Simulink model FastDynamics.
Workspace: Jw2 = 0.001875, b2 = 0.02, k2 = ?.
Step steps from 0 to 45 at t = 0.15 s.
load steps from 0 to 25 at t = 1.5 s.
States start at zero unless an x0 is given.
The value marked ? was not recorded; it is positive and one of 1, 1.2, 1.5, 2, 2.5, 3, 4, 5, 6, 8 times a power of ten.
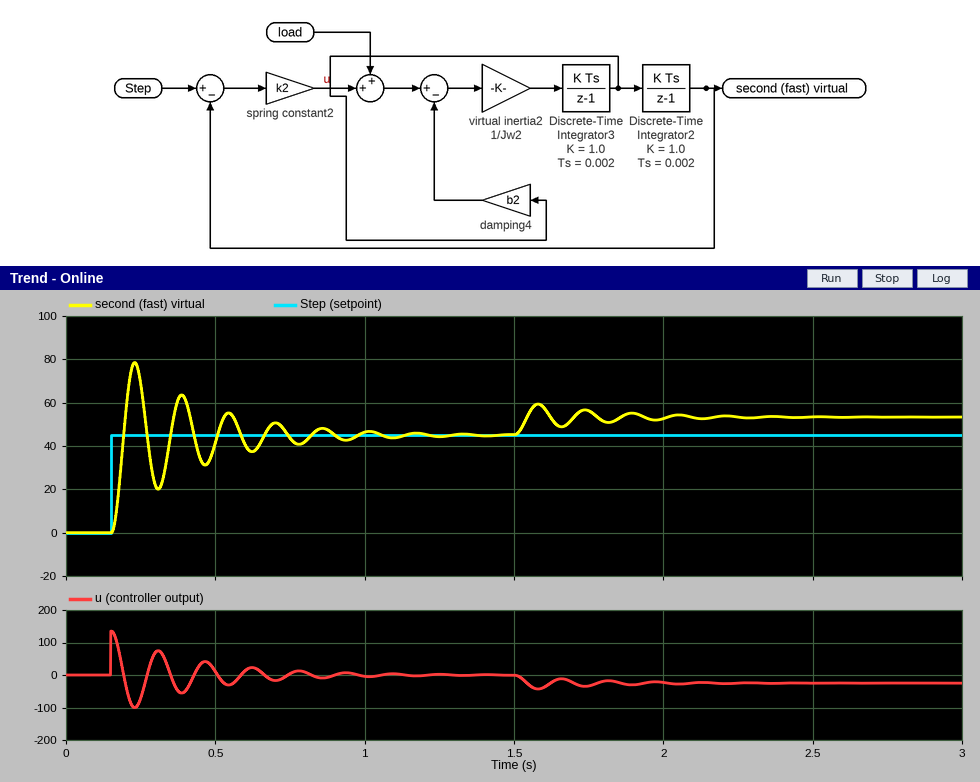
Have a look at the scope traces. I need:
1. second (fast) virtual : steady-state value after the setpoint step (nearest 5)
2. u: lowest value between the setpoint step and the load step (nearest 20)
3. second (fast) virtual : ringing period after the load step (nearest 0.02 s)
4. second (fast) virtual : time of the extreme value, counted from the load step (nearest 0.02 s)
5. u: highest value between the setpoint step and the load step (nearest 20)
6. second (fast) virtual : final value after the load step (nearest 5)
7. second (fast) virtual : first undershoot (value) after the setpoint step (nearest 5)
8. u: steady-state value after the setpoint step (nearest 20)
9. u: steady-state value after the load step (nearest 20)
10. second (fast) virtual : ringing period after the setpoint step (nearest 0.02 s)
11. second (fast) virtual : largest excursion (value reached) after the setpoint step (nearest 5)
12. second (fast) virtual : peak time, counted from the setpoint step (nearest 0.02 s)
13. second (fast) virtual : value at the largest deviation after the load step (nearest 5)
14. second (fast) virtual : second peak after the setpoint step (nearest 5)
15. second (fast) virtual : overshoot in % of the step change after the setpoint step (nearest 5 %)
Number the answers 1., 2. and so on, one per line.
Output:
1. 45
2. -100
3. 0.16 s
4. 0.08 s
5. 140
6. 55
7. 20
8. 0
9. -20
10. 0.16 s
11. 80
12. 0.08 s
13. 60
14. 65
15. 75 %
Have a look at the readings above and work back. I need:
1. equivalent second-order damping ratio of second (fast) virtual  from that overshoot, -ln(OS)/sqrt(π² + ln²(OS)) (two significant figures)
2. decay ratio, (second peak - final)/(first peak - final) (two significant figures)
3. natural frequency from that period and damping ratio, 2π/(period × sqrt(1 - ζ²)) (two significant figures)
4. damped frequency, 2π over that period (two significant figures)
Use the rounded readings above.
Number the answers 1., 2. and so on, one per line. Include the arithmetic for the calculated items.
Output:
1. ln(0.75) = -0.288; 0.288 / sqrt(9.870 + 0.083) = 0.091
2. (65 - 45) / (80 - 45) = 0.57
3. 2π / (0.16 × sqrt(1 - 0.091²)) = 39 rad/s
4. 2π / 0.16 = 39 rad/s
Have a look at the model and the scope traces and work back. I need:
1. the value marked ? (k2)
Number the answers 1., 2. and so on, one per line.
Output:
1. 3
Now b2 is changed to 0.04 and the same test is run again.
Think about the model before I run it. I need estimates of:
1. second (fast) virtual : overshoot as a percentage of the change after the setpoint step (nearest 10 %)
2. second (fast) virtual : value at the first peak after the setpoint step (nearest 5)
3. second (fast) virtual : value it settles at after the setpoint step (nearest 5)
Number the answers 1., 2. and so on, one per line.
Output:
1. 50 %
2. 65
3. 45
